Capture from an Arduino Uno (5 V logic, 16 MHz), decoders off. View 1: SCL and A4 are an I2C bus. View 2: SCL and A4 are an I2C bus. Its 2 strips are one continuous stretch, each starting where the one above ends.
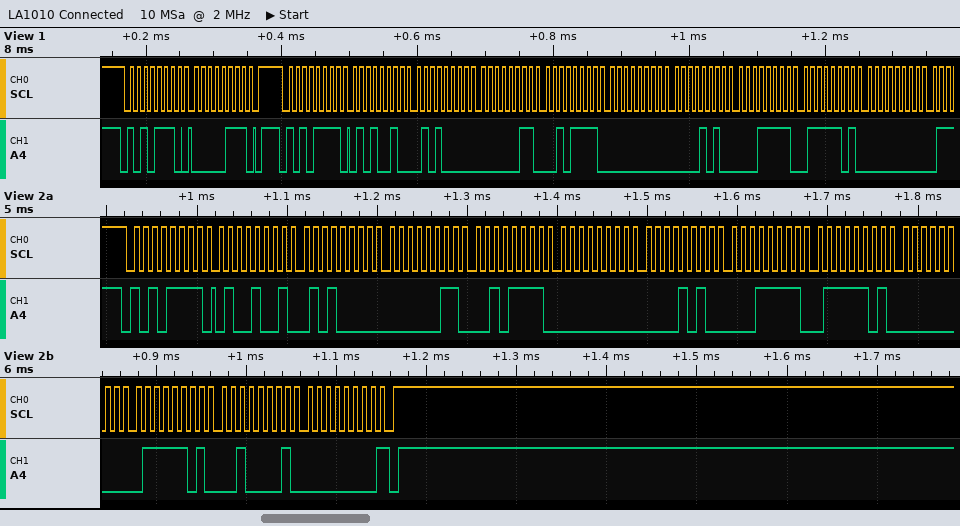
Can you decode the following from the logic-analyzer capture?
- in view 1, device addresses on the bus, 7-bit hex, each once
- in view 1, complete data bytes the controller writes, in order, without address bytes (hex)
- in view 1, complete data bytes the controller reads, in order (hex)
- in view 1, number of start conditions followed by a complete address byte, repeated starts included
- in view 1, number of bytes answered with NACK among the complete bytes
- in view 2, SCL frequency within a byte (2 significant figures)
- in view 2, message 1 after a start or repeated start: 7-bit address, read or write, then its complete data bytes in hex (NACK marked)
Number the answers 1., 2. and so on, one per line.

1. 0x57
2. 07
3. 52 50 03 2F 00 0A 1F 7D 00
4. 2
5. 0
6. 100 kHz
7. 0x57 read: 49 50 03 2F 00 0A 1F 7D 00 7D 21 00 NACK
